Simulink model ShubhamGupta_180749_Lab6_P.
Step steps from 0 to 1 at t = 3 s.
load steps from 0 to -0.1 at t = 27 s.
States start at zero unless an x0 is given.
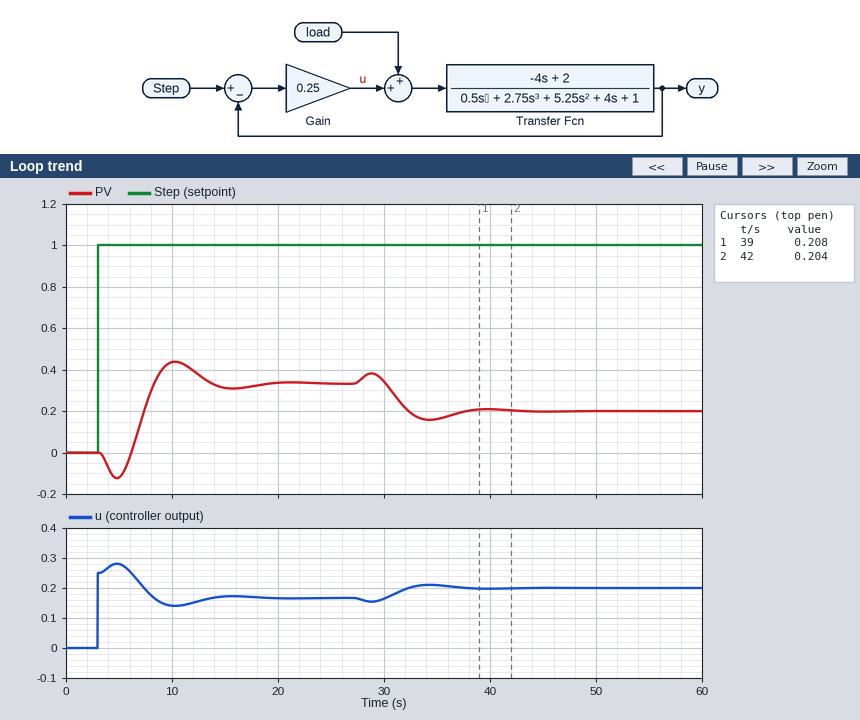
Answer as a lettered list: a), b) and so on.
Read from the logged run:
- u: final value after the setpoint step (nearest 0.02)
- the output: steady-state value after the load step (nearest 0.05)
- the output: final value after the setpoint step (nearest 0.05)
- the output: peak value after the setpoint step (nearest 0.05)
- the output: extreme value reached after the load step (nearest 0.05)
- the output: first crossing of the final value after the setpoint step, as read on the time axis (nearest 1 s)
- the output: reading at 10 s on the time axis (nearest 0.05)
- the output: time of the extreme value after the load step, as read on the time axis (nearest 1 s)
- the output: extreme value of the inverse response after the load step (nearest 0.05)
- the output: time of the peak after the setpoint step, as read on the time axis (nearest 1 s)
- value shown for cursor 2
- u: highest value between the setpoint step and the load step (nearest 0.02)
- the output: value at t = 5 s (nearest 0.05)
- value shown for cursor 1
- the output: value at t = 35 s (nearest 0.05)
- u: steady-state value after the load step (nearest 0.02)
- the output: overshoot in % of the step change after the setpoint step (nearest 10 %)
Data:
a) 0.16
b) 0.20
c) 0.35
d) 0.45
e) 0.15
f) 8 s
g) 0.45
h) 34 s
i) 0.40
j) 10 s
k) 0.204
l) 0.28
m) -0.10
n) 0.208
o) 0.15
p) 0.20
q) 30 %
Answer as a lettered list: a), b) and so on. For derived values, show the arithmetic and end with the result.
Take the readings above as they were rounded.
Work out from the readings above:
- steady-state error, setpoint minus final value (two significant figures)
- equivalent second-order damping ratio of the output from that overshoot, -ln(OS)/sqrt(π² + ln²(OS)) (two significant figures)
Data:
a) 1 - 0.35 = 0.65
b) ln(0.3) = -1.204; 1.204 / sqrt(9.870 + 1.450) = 0.36
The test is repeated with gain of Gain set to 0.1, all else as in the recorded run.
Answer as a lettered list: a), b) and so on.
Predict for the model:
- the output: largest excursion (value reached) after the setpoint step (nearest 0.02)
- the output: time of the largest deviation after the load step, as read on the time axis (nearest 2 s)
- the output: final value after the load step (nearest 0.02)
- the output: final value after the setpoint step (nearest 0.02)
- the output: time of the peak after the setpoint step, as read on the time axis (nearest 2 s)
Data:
a) 0.18
b) 36 s
c) 0.00
d) 0.16
e) 12 s
